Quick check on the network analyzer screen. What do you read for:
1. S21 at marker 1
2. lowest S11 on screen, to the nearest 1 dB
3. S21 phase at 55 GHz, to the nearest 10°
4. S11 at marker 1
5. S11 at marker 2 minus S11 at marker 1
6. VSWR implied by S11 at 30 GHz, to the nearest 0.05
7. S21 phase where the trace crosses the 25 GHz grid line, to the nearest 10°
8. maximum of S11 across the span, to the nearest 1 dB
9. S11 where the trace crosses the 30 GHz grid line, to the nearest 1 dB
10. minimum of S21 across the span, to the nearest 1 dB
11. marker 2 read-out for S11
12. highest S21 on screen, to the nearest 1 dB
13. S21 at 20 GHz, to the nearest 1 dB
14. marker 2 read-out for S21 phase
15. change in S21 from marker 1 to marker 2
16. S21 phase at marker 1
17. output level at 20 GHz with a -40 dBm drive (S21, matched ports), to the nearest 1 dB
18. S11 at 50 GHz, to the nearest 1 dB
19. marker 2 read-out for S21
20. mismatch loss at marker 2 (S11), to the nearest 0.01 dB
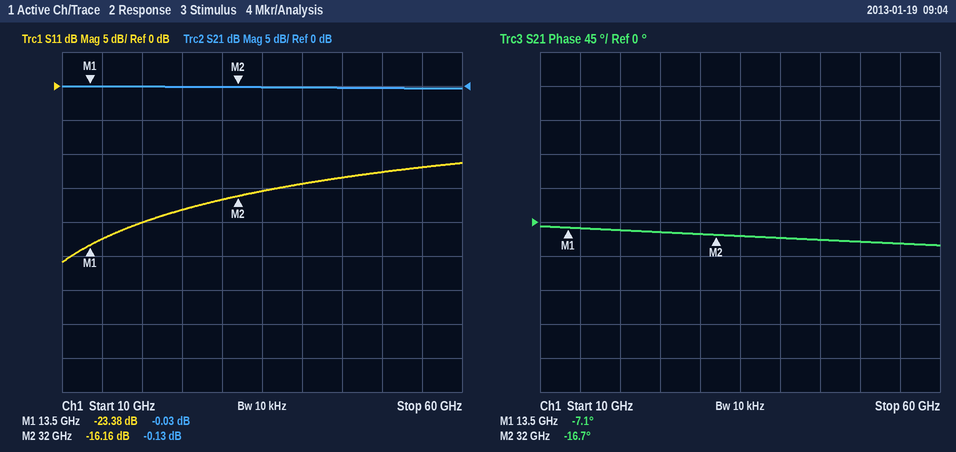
-0.03 dB
-26 dB
-30°
-23.38 dB
7.22 dB
1.35
-10°
-11 dB
-17 dB
0 dB
-16.16 dB
0 dB
0 dB
-16.7°
-0.10 dB
-7.1°
-40 dBm
-13 dB
-0.13 dB
0.11 dB
